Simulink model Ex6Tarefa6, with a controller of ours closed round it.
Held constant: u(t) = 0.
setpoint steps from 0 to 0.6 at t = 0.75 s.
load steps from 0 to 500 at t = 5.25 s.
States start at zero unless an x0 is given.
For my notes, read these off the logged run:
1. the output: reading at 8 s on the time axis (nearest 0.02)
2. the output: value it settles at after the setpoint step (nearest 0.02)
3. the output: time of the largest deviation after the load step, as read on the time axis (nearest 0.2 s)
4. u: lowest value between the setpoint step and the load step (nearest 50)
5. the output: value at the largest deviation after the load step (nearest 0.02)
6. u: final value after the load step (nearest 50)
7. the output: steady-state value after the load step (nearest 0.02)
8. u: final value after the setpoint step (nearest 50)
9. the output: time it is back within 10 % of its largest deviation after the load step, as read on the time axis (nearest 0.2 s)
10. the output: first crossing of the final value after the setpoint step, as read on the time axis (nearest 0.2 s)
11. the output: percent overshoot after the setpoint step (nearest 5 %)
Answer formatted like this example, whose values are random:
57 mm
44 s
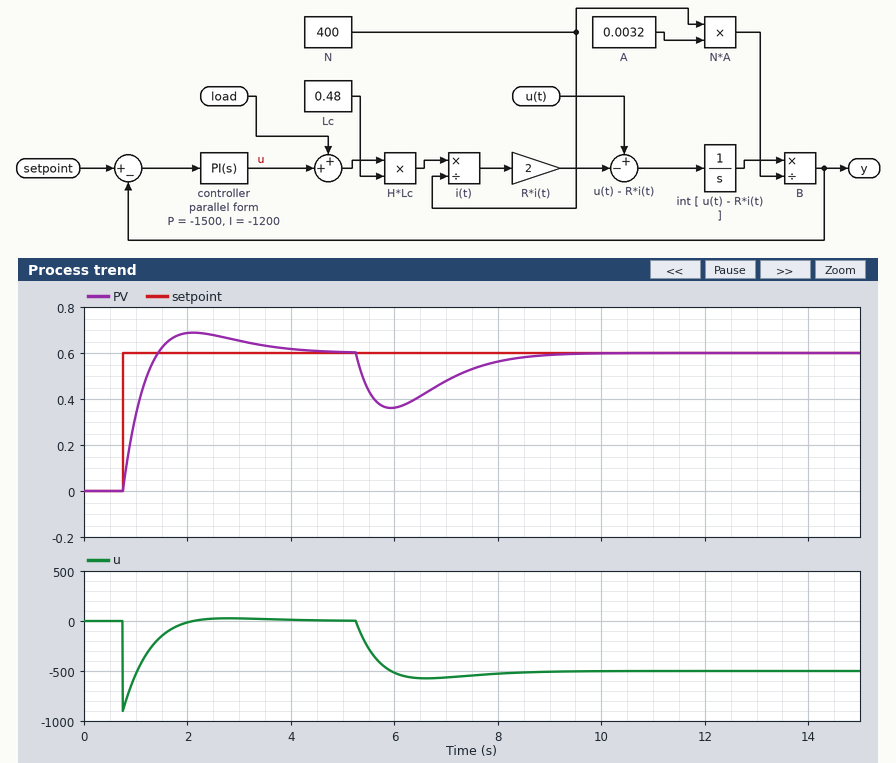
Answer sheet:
0.56
0.60
6.0 s
-900
0.36
-500
0.60
0
8.4 s
1.4 s
15 %
